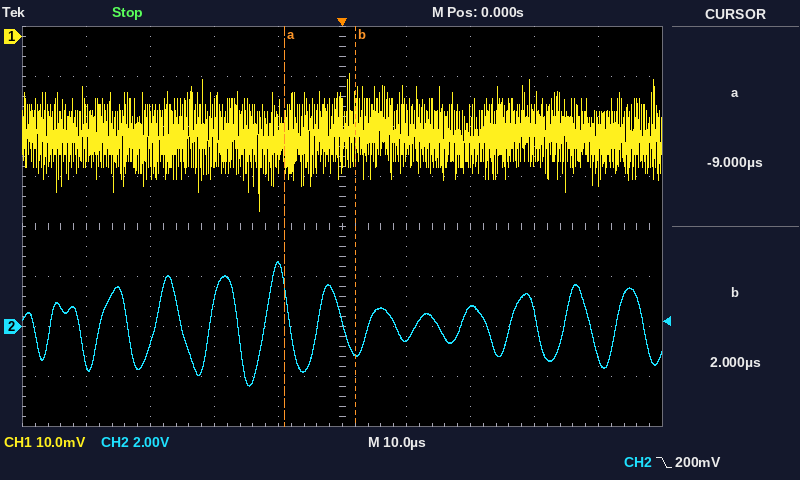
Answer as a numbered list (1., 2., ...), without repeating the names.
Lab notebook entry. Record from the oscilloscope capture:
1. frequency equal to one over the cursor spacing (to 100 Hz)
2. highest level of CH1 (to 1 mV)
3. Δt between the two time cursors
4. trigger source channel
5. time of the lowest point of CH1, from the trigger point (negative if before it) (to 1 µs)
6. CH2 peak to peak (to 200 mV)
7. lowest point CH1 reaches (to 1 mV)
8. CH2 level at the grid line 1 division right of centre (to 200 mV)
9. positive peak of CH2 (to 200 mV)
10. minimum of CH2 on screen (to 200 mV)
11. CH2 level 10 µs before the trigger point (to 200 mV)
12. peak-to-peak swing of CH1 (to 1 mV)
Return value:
1. 90.9 kHz
2. -7 mV
3. 11 µs
4. CH2
5. -13 µs
6. 5.0 V
7. -35 mV
8. -600 mV
9. 2.6 V
10. -2.4 V
11. 2.4 V
12. 28 mV
